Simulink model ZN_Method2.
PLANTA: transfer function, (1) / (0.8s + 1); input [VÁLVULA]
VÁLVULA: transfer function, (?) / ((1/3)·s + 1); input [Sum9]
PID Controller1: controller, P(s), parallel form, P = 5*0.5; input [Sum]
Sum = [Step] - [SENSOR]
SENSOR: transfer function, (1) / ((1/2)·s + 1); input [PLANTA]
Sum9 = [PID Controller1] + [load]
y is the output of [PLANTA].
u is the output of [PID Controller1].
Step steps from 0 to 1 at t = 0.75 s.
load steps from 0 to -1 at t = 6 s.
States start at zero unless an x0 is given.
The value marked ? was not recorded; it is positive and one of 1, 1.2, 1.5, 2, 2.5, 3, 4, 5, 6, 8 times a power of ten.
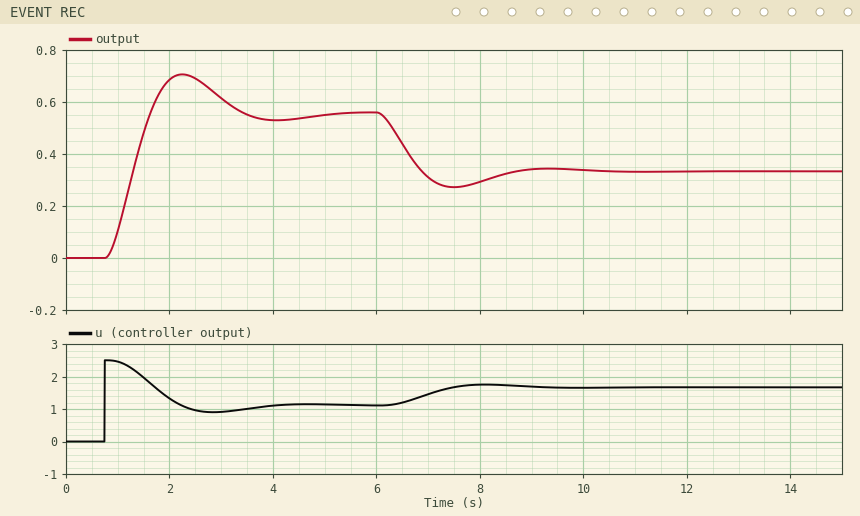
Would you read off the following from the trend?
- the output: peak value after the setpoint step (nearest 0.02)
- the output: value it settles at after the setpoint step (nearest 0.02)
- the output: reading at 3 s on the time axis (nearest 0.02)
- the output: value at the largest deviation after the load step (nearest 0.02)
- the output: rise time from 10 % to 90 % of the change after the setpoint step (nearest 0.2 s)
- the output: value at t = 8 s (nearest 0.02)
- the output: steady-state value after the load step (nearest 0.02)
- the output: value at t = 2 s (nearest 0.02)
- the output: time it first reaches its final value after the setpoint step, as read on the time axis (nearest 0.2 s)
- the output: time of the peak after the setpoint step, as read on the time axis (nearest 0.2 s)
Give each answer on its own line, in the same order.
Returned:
0.70
0.56
0.62
0.28
0.6 s
0.30
0.34
0.68
1.6 s
2.2 s
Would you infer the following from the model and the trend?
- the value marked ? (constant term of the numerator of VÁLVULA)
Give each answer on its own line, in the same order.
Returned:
0.5
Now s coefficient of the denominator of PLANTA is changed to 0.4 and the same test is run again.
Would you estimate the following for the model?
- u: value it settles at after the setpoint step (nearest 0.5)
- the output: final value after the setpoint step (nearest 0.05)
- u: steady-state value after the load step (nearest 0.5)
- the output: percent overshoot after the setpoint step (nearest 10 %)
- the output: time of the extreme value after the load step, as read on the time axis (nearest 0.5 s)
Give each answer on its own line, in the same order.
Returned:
1.0
0.55
1.5
40 %
7.0 s
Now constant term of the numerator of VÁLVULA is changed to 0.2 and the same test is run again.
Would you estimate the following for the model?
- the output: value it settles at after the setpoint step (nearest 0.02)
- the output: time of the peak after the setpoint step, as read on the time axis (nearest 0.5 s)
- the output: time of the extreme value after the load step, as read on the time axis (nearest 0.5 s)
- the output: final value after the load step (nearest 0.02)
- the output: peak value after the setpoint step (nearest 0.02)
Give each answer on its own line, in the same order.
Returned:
0.34
3.0 s
8.0 s
0.20
0.36
